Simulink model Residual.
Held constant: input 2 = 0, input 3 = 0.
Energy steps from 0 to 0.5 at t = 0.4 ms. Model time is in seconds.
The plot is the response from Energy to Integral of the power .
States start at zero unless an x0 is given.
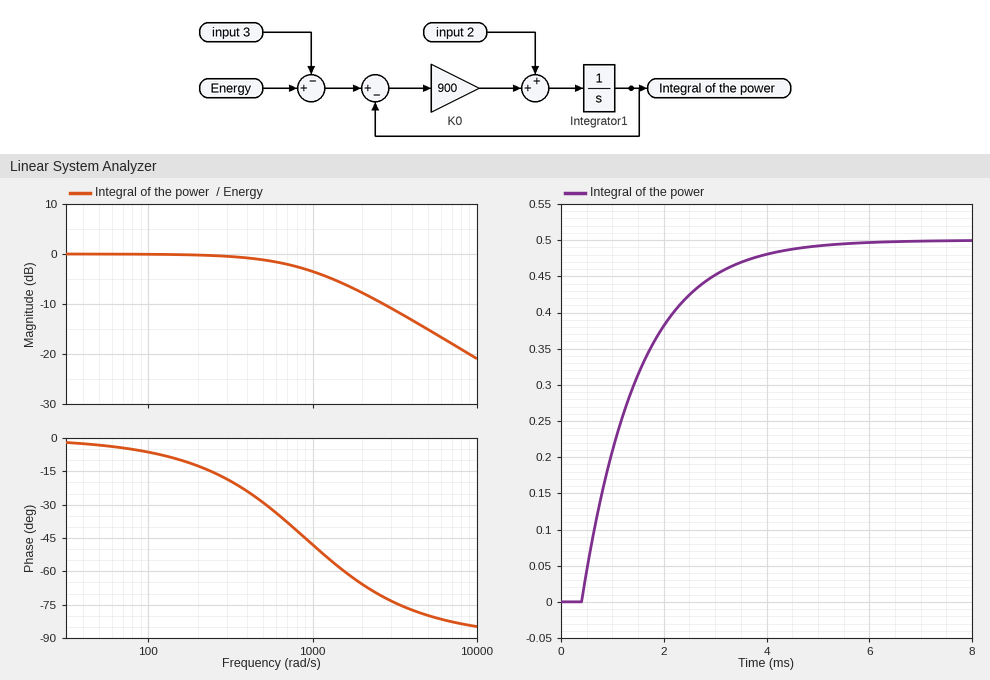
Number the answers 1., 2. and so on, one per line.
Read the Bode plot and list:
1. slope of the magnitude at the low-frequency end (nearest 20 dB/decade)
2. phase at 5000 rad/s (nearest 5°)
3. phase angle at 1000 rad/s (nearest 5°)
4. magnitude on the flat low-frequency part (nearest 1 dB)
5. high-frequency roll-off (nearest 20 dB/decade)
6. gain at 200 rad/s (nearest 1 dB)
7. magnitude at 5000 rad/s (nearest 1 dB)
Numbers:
1. 0 dB/decade
2. -80°
3. -50°
4. 0 dB
5. -20 dB/decade
6. 0 dB
7. -15 dB
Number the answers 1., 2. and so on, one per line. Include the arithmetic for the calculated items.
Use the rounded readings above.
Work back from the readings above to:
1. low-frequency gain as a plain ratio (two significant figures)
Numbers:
1. 10^(0 / 20) = 1.0
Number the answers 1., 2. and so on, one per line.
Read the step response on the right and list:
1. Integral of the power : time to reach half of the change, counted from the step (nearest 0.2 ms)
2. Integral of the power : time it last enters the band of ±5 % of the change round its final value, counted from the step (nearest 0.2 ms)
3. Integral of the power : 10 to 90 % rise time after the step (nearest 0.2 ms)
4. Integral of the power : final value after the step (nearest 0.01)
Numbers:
1. 0.8 ms
2. 3.4 ms
3. 2.4 ms
4. 0.50
